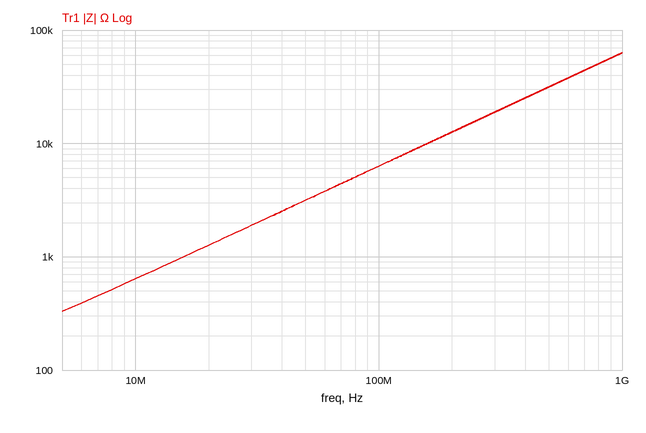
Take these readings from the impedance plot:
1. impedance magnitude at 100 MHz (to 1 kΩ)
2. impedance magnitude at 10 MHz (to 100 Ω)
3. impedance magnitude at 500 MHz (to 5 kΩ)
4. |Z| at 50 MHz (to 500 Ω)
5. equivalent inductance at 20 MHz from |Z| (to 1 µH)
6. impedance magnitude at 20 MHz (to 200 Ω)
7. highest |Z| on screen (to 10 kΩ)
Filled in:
6 kΩ
600 Ω
30 kΩ
3.0 kΩ
10 µH
1.2 kΩ
60 kΩ
